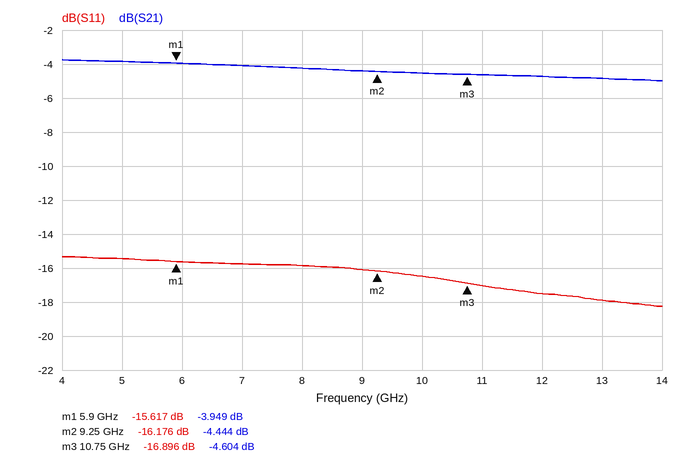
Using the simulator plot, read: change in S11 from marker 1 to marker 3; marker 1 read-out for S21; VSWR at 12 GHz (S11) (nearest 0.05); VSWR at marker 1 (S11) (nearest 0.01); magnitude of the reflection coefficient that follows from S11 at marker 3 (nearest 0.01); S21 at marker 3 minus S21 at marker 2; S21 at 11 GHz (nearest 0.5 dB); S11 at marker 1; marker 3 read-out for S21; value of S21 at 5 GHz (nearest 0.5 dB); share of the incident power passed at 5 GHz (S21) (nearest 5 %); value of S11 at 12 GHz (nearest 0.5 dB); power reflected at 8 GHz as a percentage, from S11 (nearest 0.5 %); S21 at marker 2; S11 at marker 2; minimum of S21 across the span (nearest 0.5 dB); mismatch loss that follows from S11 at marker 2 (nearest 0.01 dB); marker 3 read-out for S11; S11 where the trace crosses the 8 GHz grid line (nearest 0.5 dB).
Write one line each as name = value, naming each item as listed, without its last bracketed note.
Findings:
change in S11 from marker 1 to marker 3 = -1.279 dB
marker 1 read-out for S21 = -3.949 dB
VSWR at 12 GHz (S11) = 1.30
VSWR at marker 1 (S11) = 1.40
magnitude of the reflection coefficient that follows from S11 at marker 3 = 0.14
S21 at marker 3 minus S21 at marker 2 = -0.160 dB
S21 at 11 GHz = -4.5 dB
S11 at marker 1 = -15.617 dB
marker 3 read-out for S21 = -4.604 dB
value of S21 at 5 GHz = -4.0 dB
share of the incident power passed at 5 GHz (S21) = 40 %
value of S11 at 12 GHz = -17.5 dB
power reflected at 8 GHz as a percentage, from S11 = 2.5 %
S21 at marker 2 = -4.444 dB
S11 at marker 2 = -16.176 dB
minimum of S21 across the span = -5.0 dB
mismatch loss that follows from S11 at marker 2 = 0.11 dB
marker 3 read-out for S11 = -16.896 dB
S11 where the trace crosses the 8 GHz grid line = -16.0 dB
